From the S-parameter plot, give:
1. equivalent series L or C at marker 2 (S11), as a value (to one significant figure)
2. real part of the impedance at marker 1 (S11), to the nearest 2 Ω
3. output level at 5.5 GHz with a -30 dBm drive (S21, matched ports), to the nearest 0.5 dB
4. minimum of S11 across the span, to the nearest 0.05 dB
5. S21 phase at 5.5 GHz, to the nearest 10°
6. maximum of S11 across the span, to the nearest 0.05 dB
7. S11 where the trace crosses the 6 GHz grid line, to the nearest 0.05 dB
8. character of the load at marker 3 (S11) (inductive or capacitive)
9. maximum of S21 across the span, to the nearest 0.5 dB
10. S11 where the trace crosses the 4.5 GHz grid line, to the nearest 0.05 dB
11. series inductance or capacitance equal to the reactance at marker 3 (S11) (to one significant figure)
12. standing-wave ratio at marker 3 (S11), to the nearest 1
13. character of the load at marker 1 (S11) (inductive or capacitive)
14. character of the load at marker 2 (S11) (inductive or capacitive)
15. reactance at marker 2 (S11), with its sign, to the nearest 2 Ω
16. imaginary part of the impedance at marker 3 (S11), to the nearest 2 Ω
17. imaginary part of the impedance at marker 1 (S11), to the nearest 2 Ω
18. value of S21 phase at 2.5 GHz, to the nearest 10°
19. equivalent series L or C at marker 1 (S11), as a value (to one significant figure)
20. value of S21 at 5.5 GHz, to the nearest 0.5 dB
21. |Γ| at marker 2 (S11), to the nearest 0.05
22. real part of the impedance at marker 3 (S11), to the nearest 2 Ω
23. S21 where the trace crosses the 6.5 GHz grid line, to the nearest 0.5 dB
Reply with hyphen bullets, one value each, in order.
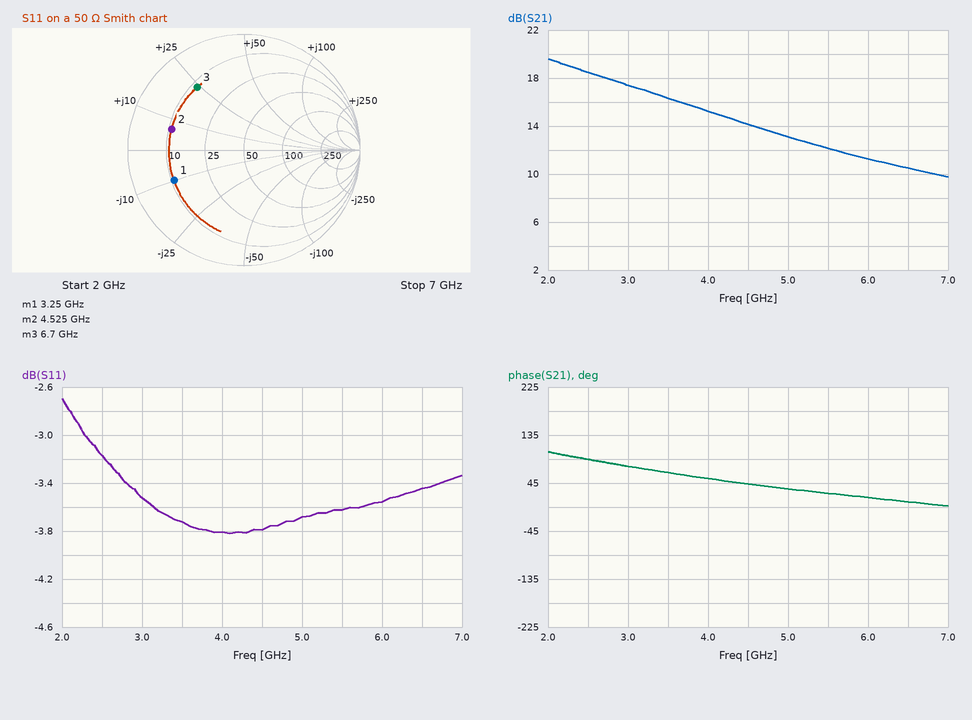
- 200 pH
- 10 Ω
- -18.0 dBm
- -3.80 dB
- 30°
- -2.70 dB
- -3.55 dB
- inductive
- 19.5 dB
- -3.80 dB
- 600 pH
- 5
- capacitive
- inductive
- +6 Ω
- +24 Ω
- -10 Ω
- 90°
- 5 pF
- 12.0 dB
- 0.65
- 12 Ω
- 10.5 dB
